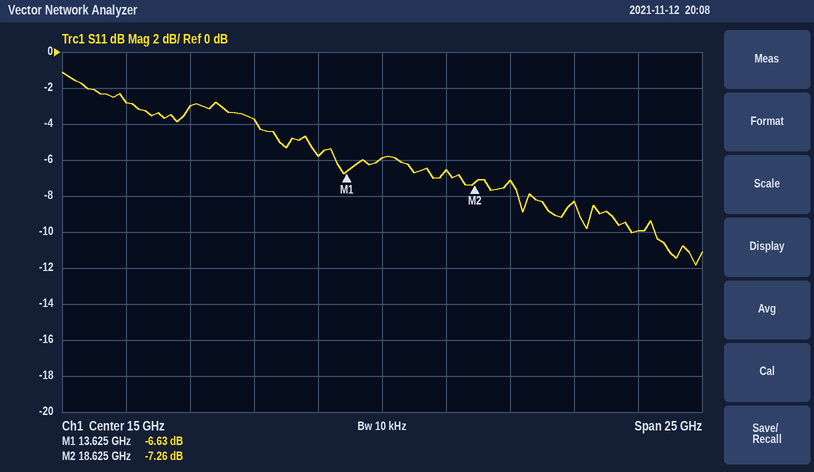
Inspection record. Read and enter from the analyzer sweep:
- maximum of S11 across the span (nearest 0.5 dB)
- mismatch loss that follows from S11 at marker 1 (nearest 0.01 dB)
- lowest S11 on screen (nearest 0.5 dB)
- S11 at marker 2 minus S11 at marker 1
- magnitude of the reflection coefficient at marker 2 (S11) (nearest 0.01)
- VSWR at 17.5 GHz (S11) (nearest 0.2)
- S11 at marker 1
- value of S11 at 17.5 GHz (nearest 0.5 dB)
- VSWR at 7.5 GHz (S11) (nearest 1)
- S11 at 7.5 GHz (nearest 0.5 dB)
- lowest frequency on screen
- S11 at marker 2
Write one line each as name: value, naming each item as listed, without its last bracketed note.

maximum of S11 across the span: -1.0 dB
mismatch loss that follows from S11 at marker 1: 1.06 dB
lowest S11 on screen: -12.0 dB
S11 at marker 2 minus S11 at marker 1: -0.63 dB
magnitude of the reflection coefficient at marker 2 (S11): 0.43
VSWR at 17.5 GHz (S11): 2.8
S11 at marker 1: -6.63 dB
value of S11 at 17.5 GHz: -6.5 dB
VSWR at 7.5 GHz (S11): 6
S11 at 7.5 GHz: -3.0 dB
lowest frequency on screen: 2.5 GHz
S11 at marker 2: -7.26 dB
